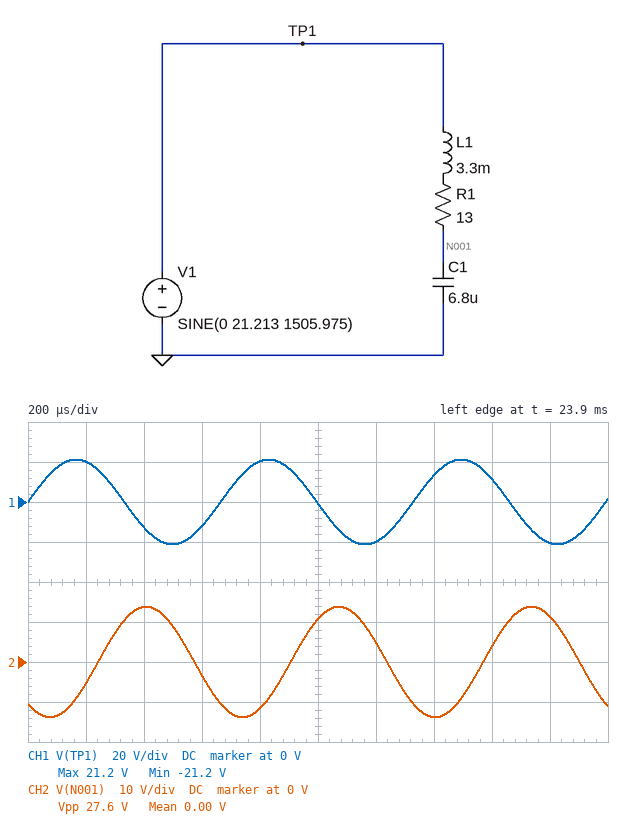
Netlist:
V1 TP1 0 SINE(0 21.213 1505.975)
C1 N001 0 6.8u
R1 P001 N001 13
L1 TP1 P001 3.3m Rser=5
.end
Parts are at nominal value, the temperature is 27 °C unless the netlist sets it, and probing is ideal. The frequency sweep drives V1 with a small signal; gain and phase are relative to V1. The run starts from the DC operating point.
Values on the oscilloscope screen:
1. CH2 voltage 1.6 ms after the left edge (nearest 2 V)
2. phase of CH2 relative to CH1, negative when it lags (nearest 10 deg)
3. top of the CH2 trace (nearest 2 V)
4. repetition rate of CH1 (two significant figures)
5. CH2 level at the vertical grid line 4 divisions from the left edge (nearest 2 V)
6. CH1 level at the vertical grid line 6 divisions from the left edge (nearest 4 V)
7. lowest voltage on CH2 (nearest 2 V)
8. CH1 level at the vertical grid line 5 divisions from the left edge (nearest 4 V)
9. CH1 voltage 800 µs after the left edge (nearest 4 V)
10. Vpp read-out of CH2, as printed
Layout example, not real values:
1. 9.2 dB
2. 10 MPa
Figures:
1. 4 V
2. -130 deg
3. 14 V
4. 1.5 kHz
5. -12 V
6. -20 V
7. -14 V
8. 0 V
9. 20 V
10. 27.6 V
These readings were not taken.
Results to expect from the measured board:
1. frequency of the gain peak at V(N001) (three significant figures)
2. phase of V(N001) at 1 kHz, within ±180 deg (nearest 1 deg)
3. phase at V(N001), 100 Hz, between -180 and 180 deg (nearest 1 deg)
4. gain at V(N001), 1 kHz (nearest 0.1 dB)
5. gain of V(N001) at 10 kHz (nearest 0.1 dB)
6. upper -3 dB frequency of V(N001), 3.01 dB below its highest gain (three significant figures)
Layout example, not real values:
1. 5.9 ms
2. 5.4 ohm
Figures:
1. 867 Hz
2. -82 deg
3. -4 deg
4. 2.2 dB
5. -38.9 dB
6. 1.26 kHz
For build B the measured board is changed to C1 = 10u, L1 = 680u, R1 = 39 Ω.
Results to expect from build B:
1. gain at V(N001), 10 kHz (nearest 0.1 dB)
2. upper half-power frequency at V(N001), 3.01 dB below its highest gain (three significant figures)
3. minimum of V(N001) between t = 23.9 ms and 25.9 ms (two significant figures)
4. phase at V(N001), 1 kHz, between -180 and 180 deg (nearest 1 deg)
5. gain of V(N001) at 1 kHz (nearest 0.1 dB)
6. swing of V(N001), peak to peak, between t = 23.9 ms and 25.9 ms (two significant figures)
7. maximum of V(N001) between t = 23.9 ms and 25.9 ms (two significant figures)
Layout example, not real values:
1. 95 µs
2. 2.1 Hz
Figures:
1. -31.6 dB
2. 375 Hz
3. -5.1 V
4. -75 deg
5. -9.1 dB
6. 10 V
7. 5.1 V
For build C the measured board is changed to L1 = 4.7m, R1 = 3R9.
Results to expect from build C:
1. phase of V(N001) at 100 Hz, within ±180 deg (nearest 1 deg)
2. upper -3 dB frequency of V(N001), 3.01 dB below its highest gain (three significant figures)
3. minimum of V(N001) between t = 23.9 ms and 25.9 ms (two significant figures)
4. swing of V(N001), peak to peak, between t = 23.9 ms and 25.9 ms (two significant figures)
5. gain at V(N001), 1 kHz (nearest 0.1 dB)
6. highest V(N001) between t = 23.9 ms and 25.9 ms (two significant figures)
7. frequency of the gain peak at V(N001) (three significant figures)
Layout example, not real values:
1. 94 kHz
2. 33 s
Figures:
1. -2 deg
2. 1.01 kHz
3. -11 V
4. 22 V
5. 6.7 dB
6. 11 V
7. 864 Hz
